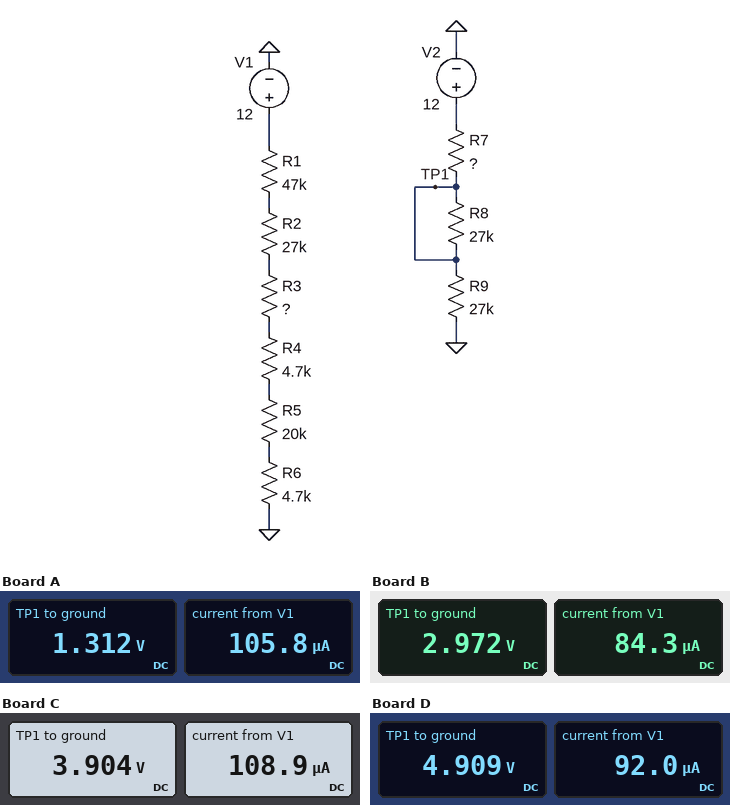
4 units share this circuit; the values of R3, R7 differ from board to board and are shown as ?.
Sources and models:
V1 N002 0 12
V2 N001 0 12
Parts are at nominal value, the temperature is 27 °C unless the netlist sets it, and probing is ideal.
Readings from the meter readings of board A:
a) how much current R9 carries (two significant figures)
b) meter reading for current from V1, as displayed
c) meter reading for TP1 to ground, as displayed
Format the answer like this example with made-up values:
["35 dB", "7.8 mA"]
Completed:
["49 µA", "105.8 µA", "1.312 V"]
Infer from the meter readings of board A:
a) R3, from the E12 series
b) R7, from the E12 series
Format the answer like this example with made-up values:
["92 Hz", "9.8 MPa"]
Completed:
["10 kΩ", "220 kΩ"]
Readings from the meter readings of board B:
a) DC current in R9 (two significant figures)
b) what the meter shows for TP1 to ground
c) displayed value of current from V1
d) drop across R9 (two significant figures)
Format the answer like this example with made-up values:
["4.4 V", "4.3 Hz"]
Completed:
["110 µA", "2.972 V", "84.3 µA", "3.0 V"]
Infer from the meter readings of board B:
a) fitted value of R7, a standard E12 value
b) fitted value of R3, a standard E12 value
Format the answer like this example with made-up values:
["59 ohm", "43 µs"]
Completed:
["82 kΩ", "39 kΩ"]
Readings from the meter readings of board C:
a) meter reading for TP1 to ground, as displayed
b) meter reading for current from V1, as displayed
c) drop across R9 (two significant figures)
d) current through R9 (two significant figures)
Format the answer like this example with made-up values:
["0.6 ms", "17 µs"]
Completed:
["3.904 V", "108.9 µA", "3.9 V", "140 µA"]
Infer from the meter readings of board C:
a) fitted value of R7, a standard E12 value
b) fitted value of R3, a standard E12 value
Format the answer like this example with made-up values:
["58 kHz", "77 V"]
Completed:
["56 kΩ", "6.8 kΩ"]
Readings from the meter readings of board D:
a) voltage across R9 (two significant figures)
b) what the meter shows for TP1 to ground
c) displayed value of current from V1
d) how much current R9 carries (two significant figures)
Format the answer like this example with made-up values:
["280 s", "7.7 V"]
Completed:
["4.9 V", "4.909 V", "92.0 µA", "180 µA"]
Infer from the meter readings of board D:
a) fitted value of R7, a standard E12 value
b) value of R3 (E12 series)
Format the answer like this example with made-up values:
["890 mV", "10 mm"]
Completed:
["39 kΩ", "27 kΩ"]
